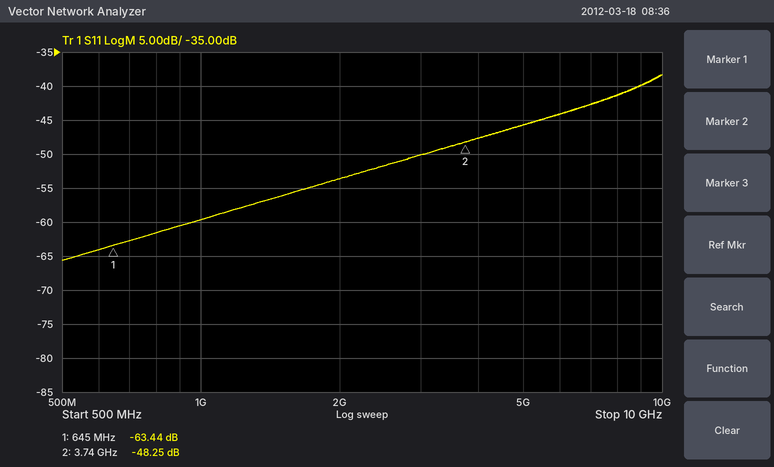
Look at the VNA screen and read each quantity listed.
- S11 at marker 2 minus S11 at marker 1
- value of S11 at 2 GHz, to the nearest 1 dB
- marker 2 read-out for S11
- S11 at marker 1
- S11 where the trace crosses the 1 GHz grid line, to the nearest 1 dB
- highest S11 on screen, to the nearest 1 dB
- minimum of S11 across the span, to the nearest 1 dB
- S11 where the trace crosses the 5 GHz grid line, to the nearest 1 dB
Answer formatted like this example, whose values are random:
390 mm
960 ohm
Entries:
15.19 dB
-54 dB
-48.25 dB
-63.44 dB
-60 dB
-38 dB
-66 dB
-46 dB
